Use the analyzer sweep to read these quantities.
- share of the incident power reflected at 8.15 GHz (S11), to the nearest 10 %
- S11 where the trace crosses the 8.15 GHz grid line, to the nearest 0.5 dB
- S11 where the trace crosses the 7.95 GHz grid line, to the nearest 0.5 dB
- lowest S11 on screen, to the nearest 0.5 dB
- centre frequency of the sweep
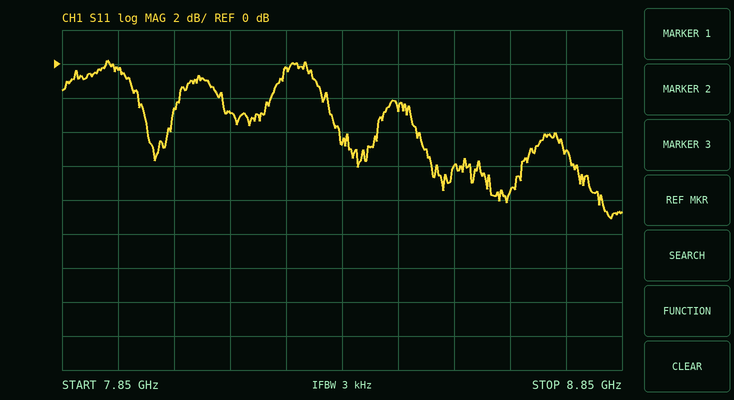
50 %
-3.0 dB
-0.5 dB
-9.0 dB
8.35 GHz
